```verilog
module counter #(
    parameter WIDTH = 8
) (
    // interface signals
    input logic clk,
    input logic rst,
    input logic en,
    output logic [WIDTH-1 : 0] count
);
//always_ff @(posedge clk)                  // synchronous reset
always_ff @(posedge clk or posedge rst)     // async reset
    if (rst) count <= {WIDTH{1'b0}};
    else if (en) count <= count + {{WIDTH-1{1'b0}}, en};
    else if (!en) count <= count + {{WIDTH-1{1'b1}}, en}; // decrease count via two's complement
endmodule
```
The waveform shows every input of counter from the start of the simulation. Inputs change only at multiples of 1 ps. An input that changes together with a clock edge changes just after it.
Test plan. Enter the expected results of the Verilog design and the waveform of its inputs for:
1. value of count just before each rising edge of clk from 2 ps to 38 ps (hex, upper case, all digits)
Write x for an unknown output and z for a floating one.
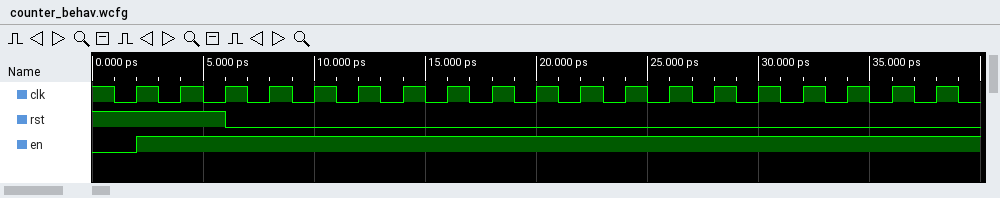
00, 00, 00, 00, 01, 02, 03, 04, 05, 06, 07, 08, 09, 0A, 0B, 0C, 0D, 0E, 0F
